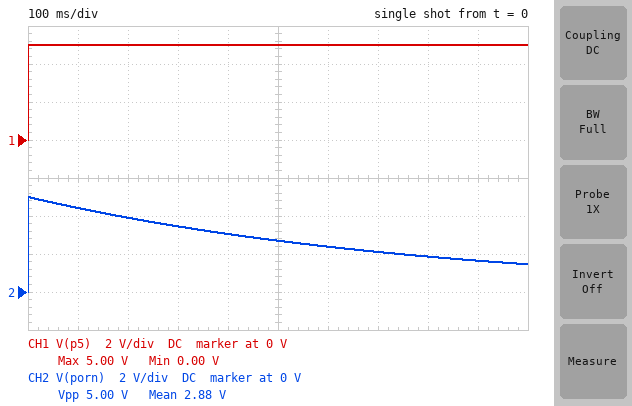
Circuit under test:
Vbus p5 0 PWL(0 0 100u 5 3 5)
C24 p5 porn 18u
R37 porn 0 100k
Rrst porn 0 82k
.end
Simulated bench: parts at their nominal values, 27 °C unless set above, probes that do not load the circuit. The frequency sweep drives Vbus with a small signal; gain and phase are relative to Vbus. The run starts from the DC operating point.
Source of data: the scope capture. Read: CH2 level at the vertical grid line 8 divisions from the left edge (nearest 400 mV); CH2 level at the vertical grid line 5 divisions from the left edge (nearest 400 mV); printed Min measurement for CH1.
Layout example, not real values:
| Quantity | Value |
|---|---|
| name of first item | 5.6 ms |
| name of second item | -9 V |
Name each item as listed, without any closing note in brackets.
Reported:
| Quantity | Value |
|---|---|
| CH2 level at the vertical grid line 8 divisions from the left edge | 2.0 V |
| CH2 level at the vertical grid line 5 divisions from the left edge | 2.8 V |
| printed Min measurement for CH1 | 0.00 V |
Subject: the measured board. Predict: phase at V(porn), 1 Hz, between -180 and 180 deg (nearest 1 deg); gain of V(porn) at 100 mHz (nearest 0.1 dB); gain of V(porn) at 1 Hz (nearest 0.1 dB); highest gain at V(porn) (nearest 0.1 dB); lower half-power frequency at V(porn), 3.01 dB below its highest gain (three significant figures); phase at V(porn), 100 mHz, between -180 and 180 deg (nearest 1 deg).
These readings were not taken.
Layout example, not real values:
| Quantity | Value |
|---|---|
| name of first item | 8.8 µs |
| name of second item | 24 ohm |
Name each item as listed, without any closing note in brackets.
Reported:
| Quantity | Value |
|---|---|
| phase at V(porn), 1 Hz, between -180 and 180 deg | 11 deg |
| gain of V(porn) at 100 mHz | -6.9 dB |
| gain of V(porn) at 1 Hz | -0.2 dB |
| highest gain at V(porn) | 0 dB |
| lower half-power frequency at V(porn), 3.01 dB below its highest gain | 196 mHz |
| phase at V(porn), 100 mHz, between -180 and 180 deg | 63 deg |
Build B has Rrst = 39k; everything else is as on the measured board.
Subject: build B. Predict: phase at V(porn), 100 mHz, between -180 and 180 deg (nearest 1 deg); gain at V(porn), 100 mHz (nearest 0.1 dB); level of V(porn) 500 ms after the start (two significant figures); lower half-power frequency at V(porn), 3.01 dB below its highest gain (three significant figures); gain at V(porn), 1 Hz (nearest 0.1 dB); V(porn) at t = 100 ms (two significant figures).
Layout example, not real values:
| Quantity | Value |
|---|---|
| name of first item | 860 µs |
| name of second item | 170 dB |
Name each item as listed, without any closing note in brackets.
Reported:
| Quantity | Value |
|---|---|
| phase at V(porn), 100 mHz, between -180 and 180 deg | 72 deg |
| gain at V(porn), 100 mHz | -10.4 dB |
| level of V(porn) 500 ms after the start | 1.9 V |
| lower half-power frequency at V(porn), 3.01 dB below its highest gain | 315 mHz |
| gain at V(porn), 1 Hz | -0.4 dB |
| V(porn) at t = 100 ms | 4.1 V |
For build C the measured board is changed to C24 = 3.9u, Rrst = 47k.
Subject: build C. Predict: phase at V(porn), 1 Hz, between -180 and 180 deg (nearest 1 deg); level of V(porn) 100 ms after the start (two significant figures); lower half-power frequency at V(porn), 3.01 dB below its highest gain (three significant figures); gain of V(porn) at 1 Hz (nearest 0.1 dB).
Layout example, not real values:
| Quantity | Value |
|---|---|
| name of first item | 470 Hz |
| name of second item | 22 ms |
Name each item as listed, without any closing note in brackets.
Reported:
| Quantity | Value |
|---|---|
| phase at V(porn), 1 Hz, between -180 and 180 deg | 52 deg |
| level of V(porn) 100 ms after the start | 2.2 V |
| lower half-power frequency at V(porn), 3.01 dB below its highest gain | 1.28 Hz |
| gain of V(porn) at 1 Hz | -4.2 dB |
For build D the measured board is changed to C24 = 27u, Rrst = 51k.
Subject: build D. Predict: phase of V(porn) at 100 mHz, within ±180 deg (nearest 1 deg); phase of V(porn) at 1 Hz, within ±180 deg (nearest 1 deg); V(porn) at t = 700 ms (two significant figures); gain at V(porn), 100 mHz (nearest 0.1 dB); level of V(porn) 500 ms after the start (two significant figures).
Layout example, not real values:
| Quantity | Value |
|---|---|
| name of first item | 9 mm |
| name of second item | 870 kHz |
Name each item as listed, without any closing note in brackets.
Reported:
| Quantity | Value |
|---|---|
| phase of V(porn) at 100 mHz, within ±180 deg | 60 deg |
| phase of V(porn) at 1 Hz, within ±180 deg | 10 deg |
| V(porn) at t = 700 ms | 2.3 V |
| gain at V(porn), 100 mHz | -6.1 dB |
| level of V(porn) 500 ms after the start | 2.9 V |
